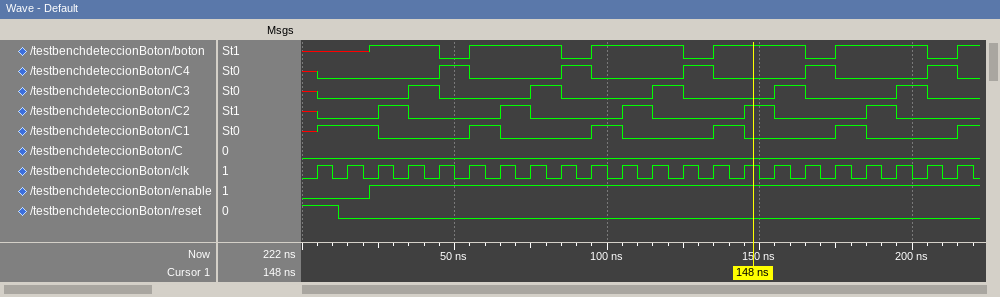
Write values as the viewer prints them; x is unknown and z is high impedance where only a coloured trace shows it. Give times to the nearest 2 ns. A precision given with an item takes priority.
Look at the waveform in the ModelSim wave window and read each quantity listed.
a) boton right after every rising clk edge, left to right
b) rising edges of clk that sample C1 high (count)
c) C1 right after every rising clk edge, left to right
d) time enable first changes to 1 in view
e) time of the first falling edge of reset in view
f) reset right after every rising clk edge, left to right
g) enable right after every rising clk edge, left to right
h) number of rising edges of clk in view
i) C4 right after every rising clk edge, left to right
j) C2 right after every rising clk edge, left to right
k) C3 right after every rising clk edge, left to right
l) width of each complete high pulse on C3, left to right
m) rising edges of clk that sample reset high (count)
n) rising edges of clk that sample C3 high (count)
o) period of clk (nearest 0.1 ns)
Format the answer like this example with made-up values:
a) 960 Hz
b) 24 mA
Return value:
a) x x 1 1 0 1 1 1 0 1 1 1 0 1 1 1 0 1 1 1 0 1
b) 6
c) 1 1 0 0 0 1 0 0 0 1 0 0 0 1 0 0 0 1 0 0 0 1
d) 22 ns
e) 12 ns
f) 1 0 0 0 0 0 0 0 0 0 0 0 0 0 0 0 0 0 0 0 0 0
g) 0 0 1 1 1 1 1 1 1 1 1 1 1 1 1 1 1 1 1 1 1 1
h) 22
i) 0 0 0 0 1 0 0 0 1 0 0 0 1 0 0 0 1 0 0 0 1 0
j) 0 0 1 0 0 0 1 0 0 0 1 0 0 0 1 0 0 0 1 0 0 0
k) 0 0 0 1 0 0 0 1 0 0 0 1 0 0 0 1 0 0 0 1 0 0
l) 10 ns, 10 ns, 10 ns, 10 ns, 10 ns
m) 1
n) 5
o) 10 ns
